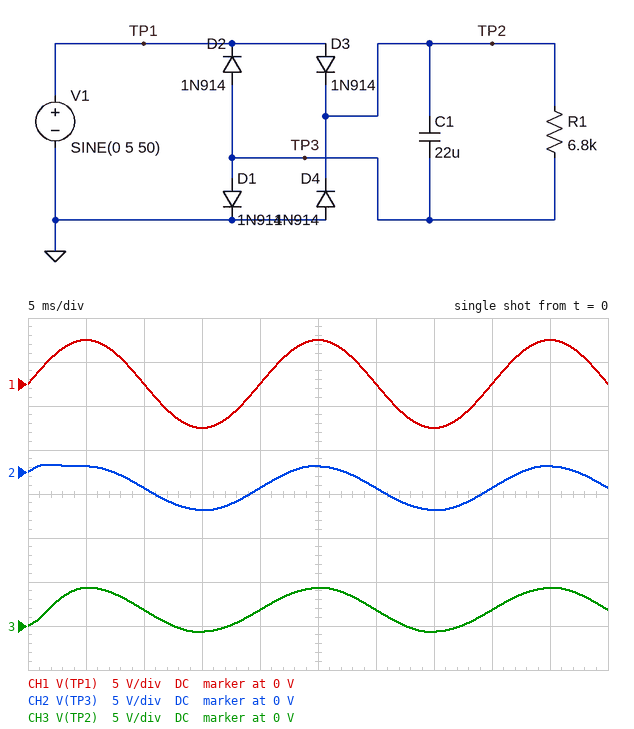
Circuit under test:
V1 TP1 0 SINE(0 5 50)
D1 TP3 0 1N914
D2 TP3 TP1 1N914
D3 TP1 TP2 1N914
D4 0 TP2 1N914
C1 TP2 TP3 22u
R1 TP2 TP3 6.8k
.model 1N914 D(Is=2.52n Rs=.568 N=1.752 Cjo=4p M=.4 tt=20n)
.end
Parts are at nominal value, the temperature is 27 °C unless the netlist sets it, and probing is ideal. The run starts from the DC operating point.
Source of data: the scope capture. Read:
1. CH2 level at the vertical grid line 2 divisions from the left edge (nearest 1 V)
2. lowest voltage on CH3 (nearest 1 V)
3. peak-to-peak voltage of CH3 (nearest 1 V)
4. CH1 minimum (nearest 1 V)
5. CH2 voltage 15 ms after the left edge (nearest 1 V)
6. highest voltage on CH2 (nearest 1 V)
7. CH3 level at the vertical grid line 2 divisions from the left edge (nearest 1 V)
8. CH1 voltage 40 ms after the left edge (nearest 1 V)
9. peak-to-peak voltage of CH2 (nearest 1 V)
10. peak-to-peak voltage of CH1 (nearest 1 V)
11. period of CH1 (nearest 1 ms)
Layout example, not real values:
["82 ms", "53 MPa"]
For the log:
["-2 V", "-1 V", "5 V", "-5 V", "-4 V", "1 V", "2 V", "0 V", "5 V", "10 V", "20 ms"]
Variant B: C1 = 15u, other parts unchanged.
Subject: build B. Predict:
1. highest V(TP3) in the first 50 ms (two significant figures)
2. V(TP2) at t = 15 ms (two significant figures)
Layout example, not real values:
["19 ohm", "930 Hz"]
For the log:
["740 mV", "-630 mV"]
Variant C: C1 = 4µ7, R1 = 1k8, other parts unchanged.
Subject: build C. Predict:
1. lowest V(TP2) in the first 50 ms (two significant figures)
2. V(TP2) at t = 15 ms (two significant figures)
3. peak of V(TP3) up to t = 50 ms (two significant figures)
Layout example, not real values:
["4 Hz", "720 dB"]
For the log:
["-670 mV", "-630 mV", "680 mV"]
